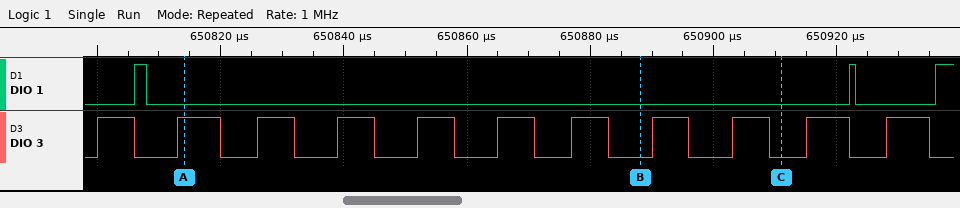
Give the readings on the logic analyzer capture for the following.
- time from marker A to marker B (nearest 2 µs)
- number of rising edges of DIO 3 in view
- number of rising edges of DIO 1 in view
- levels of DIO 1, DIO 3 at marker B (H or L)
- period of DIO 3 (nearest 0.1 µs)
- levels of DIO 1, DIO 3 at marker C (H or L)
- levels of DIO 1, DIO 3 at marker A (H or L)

74 µs
11
3
DIO 1=L, DIO 3=L
12.8 µs
DIO 1=L, DIO 3=L
DIO 1=L, DIO 3=H
